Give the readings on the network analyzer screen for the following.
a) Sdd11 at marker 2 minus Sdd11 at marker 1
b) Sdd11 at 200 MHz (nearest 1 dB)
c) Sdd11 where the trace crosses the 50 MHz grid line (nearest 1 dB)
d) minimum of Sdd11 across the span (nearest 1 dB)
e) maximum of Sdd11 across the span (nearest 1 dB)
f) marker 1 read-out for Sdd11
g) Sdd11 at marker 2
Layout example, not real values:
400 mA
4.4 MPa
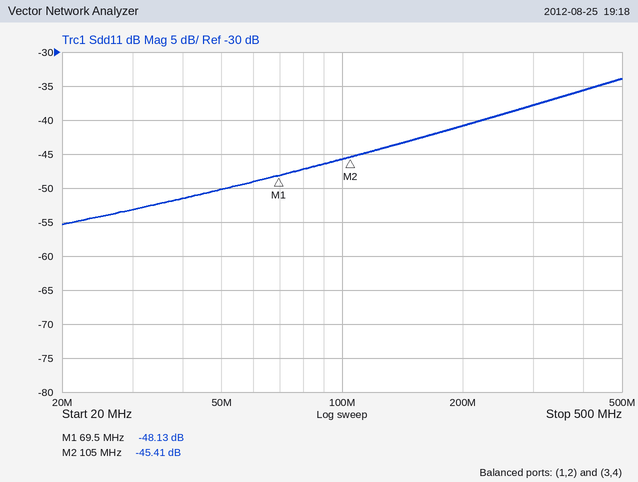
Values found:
2.72 dB
-41 dB
-50 dB
-55 dB
-34 dB
-48.13 dB
-45.41 dB
